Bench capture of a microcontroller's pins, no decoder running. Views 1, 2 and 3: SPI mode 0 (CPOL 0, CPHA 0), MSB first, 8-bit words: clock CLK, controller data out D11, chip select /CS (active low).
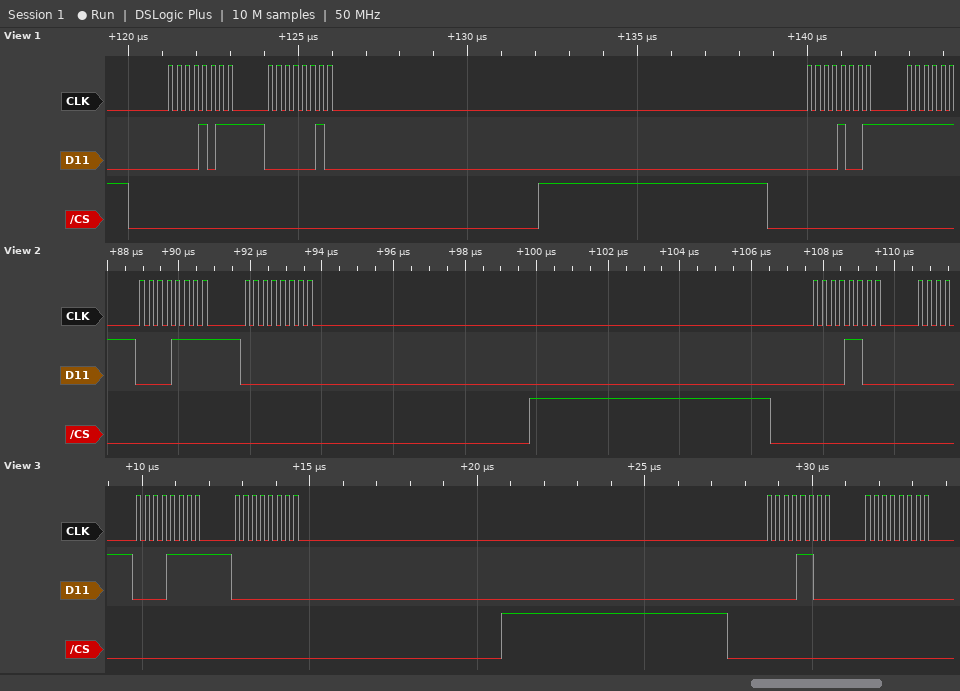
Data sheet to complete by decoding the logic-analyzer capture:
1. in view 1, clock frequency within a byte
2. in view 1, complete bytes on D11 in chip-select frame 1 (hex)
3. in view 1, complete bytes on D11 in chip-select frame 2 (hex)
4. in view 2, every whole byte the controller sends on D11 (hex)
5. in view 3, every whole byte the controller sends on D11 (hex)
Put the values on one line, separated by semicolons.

4 MHz; 0B 02; 09; 0F 00 0C; 0F 00 0C 00
